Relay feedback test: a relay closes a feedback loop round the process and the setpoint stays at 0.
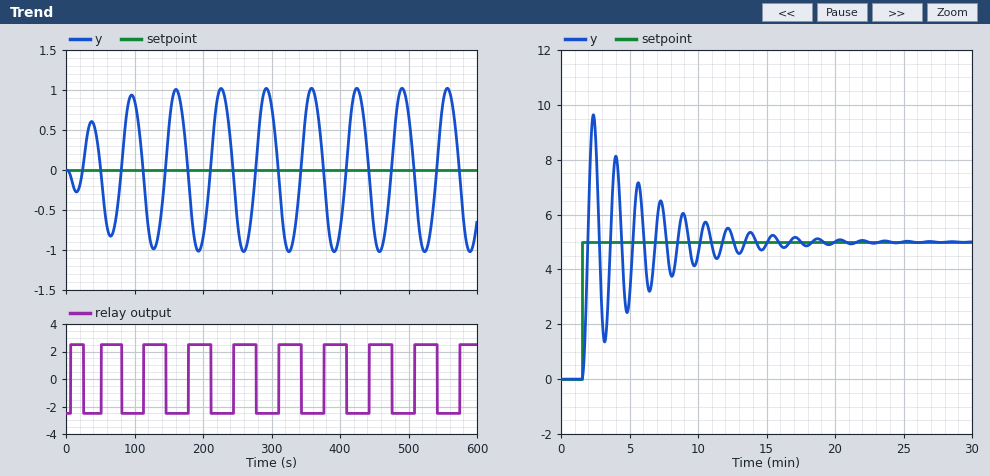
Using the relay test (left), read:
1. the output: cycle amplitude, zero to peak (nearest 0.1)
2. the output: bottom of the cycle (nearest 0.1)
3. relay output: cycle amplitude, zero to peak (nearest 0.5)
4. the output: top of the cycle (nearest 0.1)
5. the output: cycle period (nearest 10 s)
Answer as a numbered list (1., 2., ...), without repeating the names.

1. 1.0
2. -1.0
3. 2.5
4. 1.0
5. 70 s
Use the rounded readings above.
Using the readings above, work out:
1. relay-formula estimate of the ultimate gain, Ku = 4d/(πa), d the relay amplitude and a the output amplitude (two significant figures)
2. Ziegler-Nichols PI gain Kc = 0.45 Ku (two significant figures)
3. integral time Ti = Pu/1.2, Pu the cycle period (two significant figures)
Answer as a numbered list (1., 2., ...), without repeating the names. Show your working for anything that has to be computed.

1. 4 × 2.5 / (π × 1) = 3.2
2. 0.45 × 3.2 = 1.4
3. 70 / 1.2 = 58 s
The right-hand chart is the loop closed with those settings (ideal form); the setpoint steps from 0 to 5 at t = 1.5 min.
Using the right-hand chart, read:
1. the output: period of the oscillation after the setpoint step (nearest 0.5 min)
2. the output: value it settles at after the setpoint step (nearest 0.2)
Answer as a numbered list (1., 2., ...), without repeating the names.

1. 1.5 min
2. 5.0
